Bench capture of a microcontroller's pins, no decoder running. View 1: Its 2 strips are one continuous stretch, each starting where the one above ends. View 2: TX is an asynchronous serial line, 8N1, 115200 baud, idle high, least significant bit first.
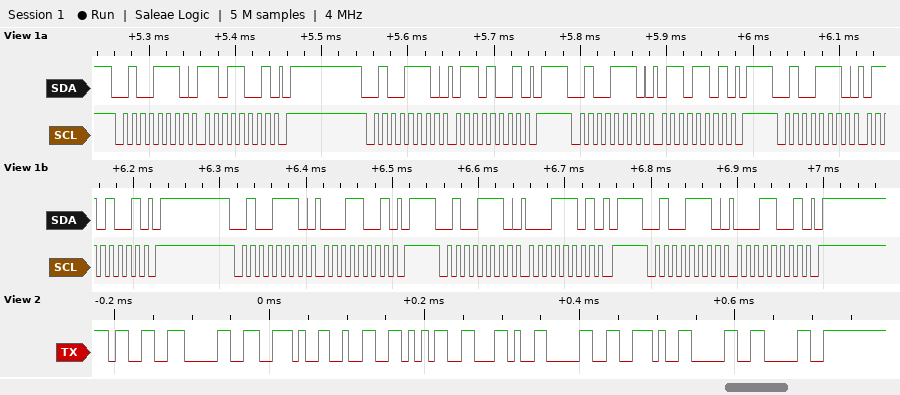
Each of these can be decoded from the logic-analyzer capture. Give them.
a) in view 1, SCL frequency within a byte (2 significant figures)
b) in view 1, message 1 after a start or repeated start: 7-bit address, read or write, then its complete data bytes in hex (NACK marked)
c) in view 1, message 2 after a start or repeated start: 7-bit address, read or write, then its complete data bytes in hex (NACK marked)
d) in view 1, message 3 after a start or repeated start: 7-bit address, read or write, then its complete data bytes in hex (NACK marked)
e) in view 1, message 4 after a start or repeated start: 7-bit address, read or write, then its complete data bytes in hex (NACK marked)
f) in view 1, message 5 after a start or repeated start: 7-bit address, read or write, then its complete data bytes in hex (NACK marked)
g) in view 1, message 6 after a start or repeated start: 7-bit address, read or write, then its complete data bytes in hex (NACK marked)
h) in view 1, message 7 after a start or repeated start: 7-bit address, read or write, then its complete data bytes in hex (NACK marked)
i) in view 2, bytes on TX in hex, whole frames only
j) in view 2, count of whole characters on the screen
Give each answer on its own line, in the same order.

100 kHz
0x27 write: D9
0x27 write: 69
0x27 write: 6D
0x27 write: 69
0x27 write: 19
0x27 write: 1D
0x27 write: 19
0x33 0x30 0x2E 0x32 0x35 0x2C 0x30 0x2E 0x30 0x30
10
